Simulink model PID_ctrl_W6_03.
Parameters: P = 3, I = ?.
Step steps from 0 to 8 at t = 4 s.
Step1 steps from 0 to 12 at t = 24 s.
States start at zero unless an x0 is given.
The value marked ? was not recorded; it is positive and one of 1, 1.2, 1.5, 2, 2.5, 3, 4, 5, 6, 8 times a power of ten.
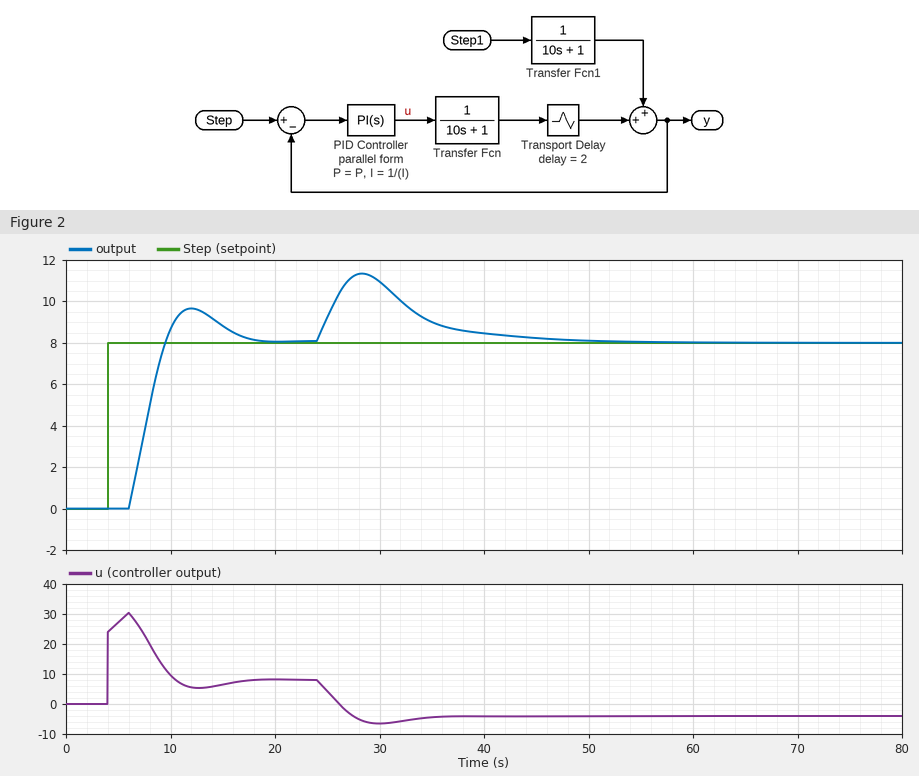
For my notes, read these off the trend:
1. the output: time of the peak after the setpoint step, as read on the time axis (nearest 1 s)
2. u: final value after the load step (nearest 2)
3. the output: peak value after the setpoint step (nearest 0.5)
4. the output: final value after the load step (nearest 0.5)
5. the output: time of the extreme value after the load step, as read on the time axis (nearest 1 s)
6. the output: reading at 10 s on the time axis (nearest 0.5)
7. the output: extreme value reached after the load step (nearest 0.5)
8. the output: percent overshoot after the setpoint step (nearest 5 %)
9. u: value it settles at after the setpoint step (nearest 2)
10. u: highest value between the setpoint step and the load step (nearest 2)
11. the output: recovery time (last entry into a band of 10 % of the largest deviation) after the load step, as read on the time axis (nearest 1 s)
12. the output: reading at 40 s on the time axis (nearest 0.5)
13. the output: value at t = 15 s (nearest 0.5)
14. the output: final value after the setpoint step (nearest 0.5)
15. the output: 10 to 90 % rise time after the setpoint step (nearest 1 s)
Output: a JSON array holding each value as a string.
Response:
["12 s", "-4", "9.5", "8.0", "28 s", "8.5", "11.5", "20 %", "8", "30", "43 s", "8.5", "9.0", "8.0", "3 s"]
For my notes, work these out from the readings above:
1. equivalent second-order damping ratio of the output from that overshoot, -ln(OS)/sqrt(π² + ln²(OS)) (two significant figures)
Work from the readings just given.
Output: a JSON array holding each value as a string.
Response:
["0.46"]
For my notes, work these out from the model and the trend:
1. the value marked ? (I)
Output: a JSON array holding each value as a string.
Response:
["2.5"]
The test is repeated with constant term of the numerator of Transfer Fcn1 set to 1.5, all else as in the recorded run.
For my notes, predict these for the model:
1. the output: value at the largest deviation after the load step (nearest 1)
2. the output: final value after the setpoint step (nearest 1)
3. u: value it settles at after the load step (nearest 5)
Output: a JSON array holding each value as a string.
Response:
["13", "8", "-10"]
